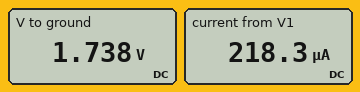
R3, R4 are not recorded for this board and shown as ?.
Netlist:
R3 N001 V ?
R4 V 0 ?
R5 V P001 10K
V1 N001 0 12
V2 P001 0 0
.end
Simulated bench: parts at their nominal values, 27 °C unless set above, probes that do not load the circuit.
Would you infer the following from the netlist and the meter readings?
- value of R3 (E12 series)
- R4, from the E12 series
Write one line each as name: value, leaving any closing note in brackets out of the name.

value of R3: 47 kΩ
R4, from the E12 series: 39 kΩ
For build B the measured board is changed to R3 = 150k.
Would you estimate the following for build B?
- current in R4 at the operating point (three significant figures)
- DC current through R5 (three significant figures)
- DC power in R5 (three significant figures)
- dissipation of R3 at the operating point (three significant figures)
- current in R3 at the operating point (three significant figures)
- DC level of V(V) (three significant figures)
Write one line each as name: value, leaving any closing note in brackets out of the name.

current in R4 at the operating point: 15.5 µA
DC current through R5: 60.5 µA
DC power in R5: 36.6 µW
dissipation of R3 at the operating point: 866 µW
current in R3 at the operating point: 76.0 µA
DC level of V(V): 605 mV
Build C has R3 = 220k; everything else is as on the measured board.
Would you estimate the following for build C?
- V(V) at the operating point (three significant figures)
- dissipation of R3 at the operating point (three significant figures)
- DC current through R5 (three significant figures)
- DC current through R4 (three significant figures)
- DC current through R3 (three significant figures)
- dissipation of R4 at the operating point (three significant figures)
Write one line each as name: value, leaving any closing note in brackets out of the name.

V(V) at the operating point: 419 mV
dissipation of R3 at the operating point: 610 µW
DC current through R5: 41.9 µA
DC current through R4: 10.7 µA
DC current through R3: 52.6 µA
dissipation of R4 at the operating point: 4.50 µW
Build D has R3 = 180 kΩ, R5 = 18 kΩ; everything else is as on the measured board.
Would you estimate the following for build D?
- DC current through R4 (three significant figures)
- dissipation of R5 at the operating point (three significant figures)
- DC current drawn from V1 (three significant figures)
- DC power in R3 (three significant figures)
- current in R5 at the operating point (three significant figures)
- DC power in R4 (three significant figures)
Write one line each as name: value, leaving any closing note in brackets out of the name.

DC current through R4: 19.7 µA
dissipation of R5 at the operating point: 32.8 µW
DC current drawn from V1: 62.4 µA
DC power in R3: 701 µW
current in R5 at the operating point: 42.7 µA
DC power in R4: 15.1 µW
